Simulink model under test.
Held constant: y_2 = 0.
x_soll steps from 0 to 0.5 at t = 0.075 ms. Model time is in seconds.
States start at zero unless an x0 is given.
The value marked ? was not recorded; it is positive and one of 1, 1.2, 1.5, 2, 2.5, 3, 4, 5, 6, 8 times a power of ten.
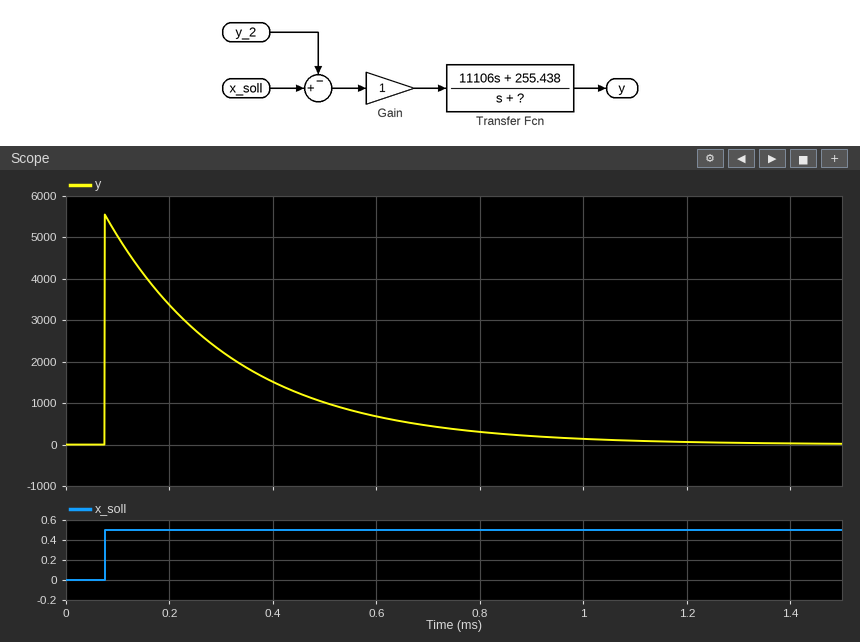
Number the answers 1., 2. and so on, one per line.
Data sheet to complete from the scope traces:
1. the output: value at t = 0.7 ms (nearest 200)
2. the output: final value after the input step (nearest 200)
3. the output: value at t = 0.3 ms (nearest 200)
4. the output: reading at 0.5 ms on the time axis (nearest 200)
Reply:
1. 400
2. 0
3. 2200
4. 1000
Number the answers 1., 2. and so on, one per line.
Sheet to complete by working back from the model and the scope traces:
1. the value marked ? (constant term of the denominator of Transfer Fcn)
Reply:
1. 4000
